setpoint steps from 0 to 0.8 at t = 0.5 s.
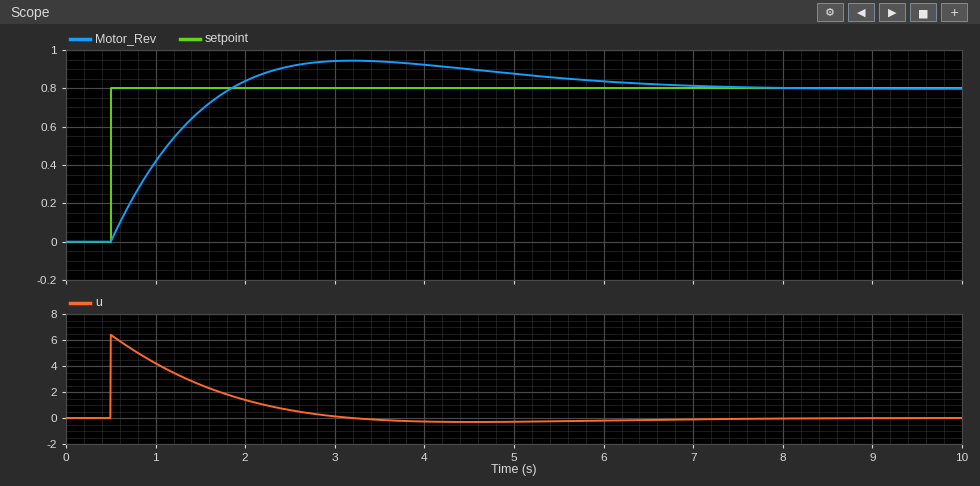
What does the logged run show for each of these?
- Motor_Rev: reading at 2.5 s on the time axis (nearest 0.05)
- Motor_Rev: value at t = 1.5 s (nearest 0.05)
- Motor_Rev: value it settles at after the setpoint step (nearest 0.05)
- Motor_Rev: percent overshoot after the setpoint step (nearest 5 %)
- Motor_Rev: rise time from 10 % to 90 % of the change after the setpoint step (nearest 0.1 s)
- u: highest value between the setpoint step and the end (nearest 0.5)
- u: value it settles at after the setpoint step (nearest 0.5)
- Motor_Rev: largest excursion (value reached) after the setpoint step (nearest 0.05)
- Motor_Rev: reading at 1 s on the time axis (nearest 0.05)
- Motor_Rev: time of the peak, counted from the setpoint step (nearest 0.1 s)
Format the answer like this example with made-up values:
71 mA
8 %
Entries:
0.90
0.70
0.80
20 %
1.0 s
6.5
0.0
0.95
0.40
2.7 s
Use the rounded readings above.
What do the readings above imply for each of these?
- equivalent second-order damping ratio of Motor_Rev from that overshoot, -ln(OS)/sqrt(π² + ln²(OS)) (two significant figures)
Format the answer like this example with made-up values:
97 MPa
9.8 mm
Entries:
0.46
